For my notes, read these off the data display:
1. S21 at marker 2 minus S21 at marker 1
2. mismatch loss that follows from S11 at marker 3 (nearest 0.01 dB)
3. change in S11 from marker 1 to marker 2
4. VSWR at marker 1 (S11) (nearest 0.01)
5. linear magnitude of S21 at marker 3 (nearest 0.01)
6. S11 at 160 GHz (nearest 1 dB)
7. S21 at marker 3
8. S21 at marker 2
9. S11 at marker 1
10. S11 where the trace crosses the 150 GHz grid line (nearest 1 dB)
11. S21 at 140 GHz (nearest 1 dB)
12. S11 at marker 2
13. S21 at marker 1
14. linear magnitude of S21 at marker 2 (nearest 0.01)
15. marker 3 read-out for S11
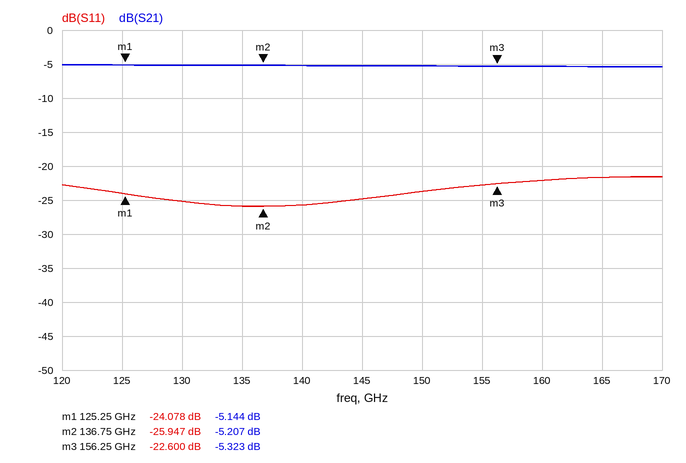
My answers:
-0.063 dB
0.02 dB
-1.869 dB
1.13
0.54
-22 dB
-5.323 dB
-5.207 dB
-24.078 dB
-24 dB
-5 dB
-25.947 dB
-5.144 dB
0.55
-22.600 dB
